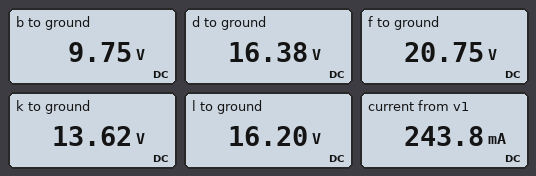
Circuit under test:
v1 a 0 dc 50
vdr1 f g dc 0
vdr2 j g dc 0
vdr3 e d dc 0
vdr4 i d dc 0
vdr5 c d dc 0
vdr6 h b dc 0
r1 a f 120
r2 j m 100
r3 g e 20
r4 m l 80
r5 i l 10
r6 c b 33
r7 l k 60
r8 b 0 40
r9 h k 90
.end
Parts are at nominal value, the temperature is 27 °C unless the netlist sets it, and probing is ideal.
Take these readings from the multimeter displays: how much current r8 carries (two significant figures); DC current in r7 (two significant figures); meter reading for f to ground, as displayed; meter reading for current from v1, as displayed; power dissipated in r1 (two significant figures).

240 mA
43 mA
20.75 V
243.8 mA
7.1 W
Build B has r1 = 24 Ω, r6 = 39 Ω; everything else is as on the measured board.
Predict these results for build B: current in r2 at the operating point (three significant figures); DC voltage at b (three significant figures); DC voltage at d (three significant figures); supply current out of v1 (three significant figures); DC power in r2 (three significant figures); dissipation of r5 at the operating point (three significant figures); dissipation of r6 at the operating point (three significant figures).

46.4 mA
17.7 V
31.5 V
442 mA
215 mW
18.2 mW
4.87 W
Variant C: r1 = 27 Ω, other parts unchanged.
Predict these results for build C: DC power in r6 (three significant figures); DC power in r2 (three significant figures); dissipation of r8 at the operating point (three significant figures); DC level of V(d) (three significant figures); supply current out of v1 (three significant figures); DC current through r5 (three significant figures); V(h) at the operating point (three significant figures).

4.45 W
214 mW
7.96 W
30.0 V
446 mA
32.4 mA
17.8 V
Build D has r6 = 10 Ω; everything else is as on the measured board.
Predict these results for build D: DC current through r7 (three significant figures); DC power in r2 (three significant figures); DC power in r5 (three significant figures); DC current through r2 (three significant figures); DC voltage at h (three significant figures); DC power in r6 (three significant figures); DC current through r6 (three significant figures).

17.2 mA
68.8 mW
809 µW
26.2 mA
10.7 V
623 mW
250 mA
